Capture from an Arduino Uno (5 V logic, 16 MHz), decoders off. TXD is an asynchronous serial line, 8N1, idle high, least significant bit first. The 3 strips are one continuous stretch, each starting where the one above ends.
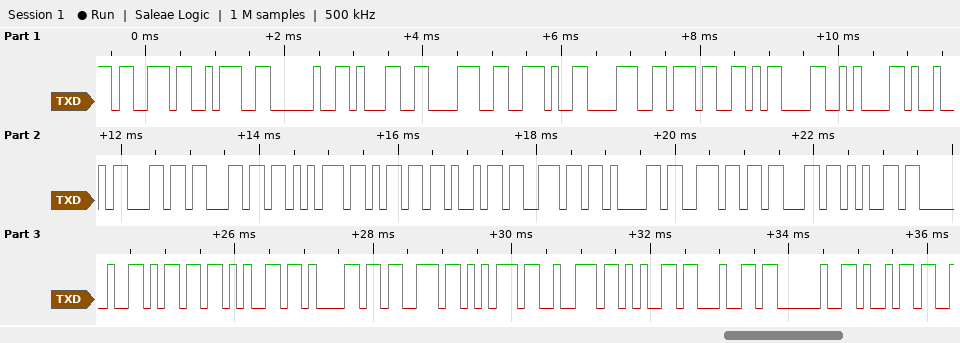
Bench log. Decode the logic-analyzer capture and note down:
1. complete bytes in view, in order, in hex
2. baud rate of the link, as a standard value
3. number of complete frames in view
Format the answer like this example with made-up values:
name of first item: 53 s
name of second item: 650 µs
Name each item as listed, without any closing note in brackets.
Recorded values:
complete bytes in view, in order, in hex: 73 3A 20 31 38 2E 38 37 0D 0A 49 6C 6C 75 6D 69 6E 61 6E 63 65 20 6D 65 61 73 75 72 65 64 20 69
baud rate of the link, as a standard value: 9600 baud
number of complete frames in view: 32
